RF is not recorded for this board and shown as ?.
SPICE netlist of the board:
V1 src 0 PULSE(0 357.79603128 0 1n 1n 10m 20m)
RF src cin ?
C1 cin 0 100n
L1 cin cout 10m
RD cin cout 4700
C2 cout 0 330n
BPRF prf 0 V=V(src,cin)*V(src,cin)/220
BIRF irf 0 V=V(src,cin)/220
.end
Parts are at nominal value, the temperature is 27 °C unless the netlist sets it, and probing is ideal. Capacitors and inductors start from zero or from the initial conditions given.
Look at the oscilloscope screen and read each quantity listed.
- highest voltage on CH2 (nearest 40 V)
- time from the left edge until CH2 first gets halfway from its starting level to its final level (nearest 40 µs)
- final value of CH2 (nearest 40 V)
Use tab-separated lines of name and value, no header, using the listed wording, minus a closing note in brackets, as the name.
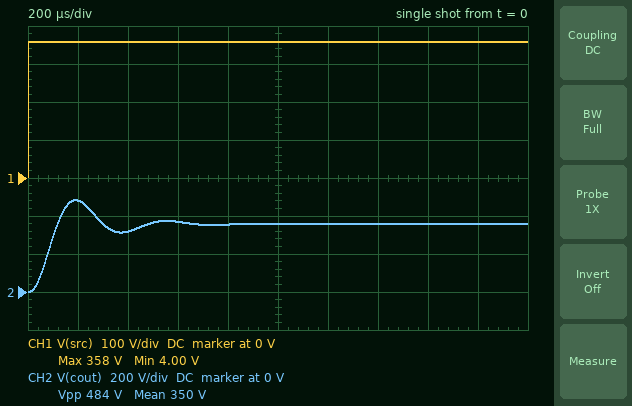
highest voltage on CH2	480 V
time from the left edge until CH2 first gets halfway from its starting level to its final level	80 µs
final value of CH2	360 V
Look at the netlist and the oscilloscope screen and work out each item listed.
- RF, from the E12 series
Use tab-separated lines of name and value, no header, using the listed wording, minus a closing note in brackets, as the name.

RF, from the E12 series	100 Ω
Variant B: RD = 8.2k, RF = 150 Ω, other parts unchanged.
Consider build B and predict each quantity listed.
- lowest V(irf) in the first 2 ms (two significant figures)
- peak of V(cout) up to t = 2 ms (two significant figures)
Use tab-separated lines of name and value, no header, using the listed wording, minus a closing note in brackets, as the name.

lowest V(irf) in the first 2 ms	-160 mV
peak of V(cout) up to t = 2 ms	420 V
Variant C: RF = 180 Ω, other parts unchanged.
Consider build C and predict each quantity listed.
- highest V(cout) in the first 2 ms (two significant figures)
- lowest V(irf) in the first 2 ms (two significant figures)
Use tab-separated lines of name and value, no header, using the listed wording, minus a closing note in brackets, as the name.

highest V(cout) in the first 2 ms	390 V
lowest V(irf) in the first 2 ms	-90 mV
